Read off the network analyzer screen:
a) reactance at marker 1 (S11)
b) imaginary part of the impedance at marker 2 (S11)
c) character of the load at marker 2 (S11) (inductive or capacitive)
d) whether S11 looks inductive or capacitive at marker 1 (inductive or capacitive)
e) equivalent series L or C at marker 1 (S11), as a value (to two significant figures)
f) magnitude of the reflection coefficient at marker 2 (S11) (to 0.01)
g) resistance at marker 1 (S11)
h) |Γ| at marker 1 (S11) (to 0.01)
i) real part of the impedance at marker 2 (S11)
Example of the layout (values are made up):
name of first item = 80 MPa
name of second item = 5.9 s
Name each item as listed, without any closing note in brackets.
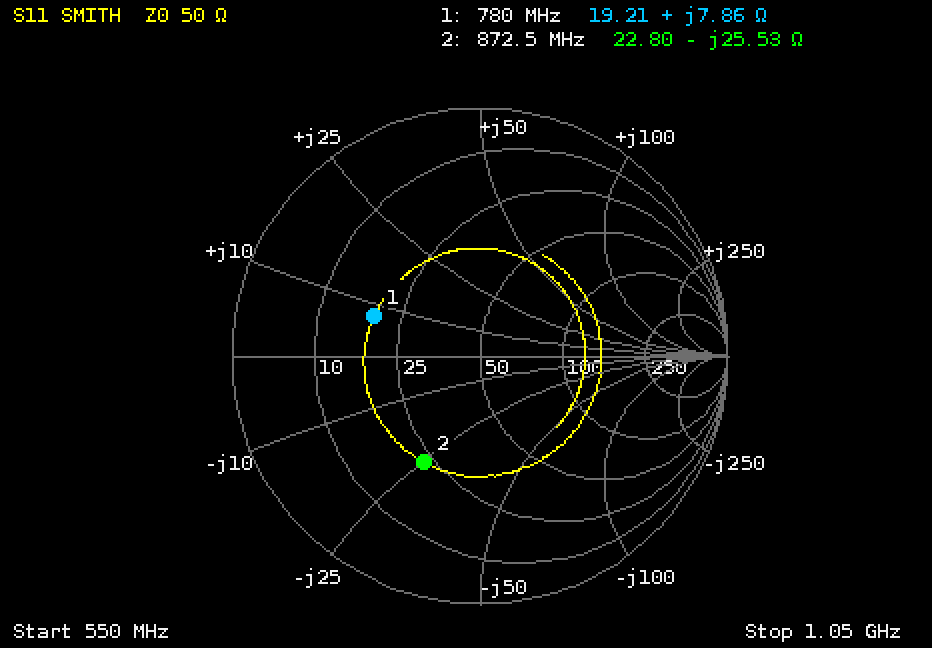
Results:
reactance at marker 1 = +7.86 Ω
imaginary part of the impedance at marker 2 = -25.53 Ω
character of the load at marker 2 (S11) = capacitive
whether S11 looks inductive or capacitive at marker 1 = inductive
equivalent series L or C at marker 1 (S11), as a value = 1.6 nH
magnitude of the reflection coefficient at marker 2 (S11) = 0.48
resistance at marker 1 = 19.21 Ω
|Γ| at marker 1 (S11) = 0.46
real part of the impedance at marker 2 = 22.80 Ω
